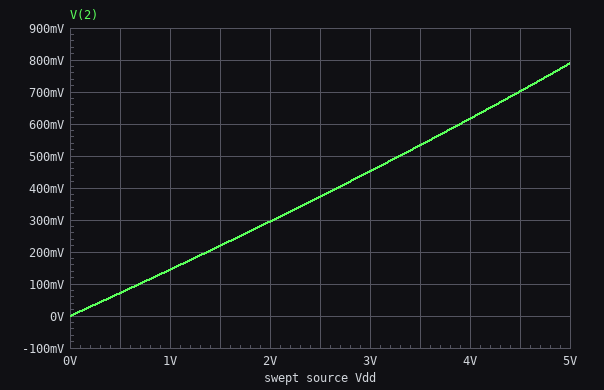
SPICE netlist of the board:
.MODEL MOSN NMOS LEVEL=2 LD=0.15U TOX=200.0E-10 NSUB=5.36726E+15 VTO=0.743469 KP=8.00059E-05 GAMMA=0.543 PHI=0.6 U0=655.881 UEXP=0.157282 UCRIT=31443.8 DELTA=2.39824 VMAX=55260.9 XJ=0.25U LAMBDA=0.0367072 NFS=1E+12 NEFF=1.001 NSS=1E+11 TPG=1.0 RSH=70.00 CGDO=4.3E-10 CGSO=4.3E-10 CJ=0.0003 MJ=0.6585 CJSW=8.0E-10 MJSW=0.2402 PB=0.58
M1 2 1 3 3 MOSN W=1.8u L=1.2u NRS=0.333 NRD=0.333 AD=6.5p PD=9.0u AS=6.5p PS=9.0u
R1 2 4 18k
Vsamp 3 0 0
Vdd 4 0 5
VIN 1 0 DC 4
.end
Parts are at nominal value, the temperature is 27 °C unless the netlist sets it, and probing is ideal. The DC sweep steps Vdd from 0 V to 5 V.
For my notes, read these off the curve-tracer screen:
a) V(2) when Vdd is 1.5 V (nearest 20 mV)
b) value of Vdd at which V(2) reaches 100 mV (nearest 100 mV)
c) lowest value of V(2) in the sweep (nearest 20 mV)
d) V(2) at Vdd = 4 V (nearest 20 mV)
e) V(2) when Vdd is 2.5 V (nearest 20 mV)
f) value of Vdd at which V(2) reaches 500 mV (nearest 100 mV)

220 mV
700 mV
0 V
620 mV
380 mV
3.3 V
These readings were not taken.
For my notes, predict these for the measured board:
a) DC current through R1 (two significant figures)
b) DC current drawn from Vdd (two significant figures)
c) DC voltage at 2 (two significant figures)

230 µA
230 µA
790 mV
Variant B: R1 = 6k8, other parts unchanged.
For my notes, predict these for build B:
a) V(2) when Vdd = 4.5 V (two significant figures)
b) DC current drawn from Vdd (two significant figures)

2.5 V
300 µA
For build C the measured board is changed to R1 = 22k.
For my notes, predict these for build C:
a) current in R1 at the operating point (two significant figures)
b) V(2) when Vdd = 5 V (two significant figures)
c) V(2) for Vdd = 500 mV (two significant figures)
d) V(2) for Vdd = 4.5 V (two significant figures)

200 µA
650 mV
60 mV
580 mV
